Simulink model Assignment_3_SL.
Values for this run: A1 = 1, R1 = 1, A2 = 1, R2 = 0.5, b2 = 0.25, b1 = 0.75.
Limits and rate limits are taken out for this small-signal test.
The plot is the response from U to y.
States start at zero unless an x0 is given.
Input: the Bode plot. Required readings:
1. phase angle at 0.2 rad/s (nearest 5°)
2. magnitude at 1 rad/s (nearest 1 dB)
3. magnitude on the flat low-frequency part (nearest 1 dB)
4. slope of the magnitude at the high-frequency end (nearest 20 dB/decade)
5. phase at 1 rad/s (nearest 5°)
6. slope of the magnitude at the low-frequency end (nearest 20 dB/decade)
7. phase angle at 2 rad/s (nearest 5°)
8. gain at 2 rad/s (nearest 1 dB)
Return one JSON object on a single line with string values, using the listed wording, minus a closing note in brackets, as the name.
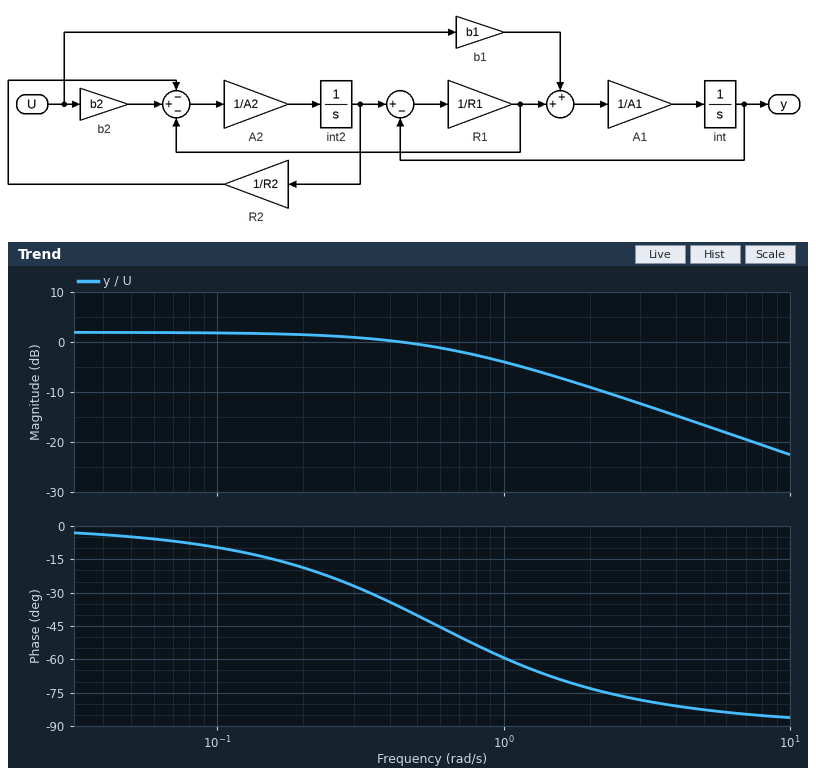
{"phase angle at 0.2 rad/s": "-20°", "magnitude at 1 rad/s": "-4 dB", "magnitude on the flat low-frequency part": "2 dB", "slope of the magnitude at the high-frequency end": "-20 dB/decade", "phase at 1 rad/s": "-60°", "slope of the magnitude at the low-frequency end": "0 dB/decade", "phase angle at 2 rad/s": "-75°", "gain at 2 rad/s": "-9 dB"}
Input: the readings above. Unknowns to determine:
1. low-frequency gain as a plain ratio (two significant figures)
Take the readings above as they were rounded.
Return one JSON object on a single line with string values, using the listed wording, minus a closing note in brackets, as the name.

{"low-frequency gain as a plain ratio": "1.3"}
